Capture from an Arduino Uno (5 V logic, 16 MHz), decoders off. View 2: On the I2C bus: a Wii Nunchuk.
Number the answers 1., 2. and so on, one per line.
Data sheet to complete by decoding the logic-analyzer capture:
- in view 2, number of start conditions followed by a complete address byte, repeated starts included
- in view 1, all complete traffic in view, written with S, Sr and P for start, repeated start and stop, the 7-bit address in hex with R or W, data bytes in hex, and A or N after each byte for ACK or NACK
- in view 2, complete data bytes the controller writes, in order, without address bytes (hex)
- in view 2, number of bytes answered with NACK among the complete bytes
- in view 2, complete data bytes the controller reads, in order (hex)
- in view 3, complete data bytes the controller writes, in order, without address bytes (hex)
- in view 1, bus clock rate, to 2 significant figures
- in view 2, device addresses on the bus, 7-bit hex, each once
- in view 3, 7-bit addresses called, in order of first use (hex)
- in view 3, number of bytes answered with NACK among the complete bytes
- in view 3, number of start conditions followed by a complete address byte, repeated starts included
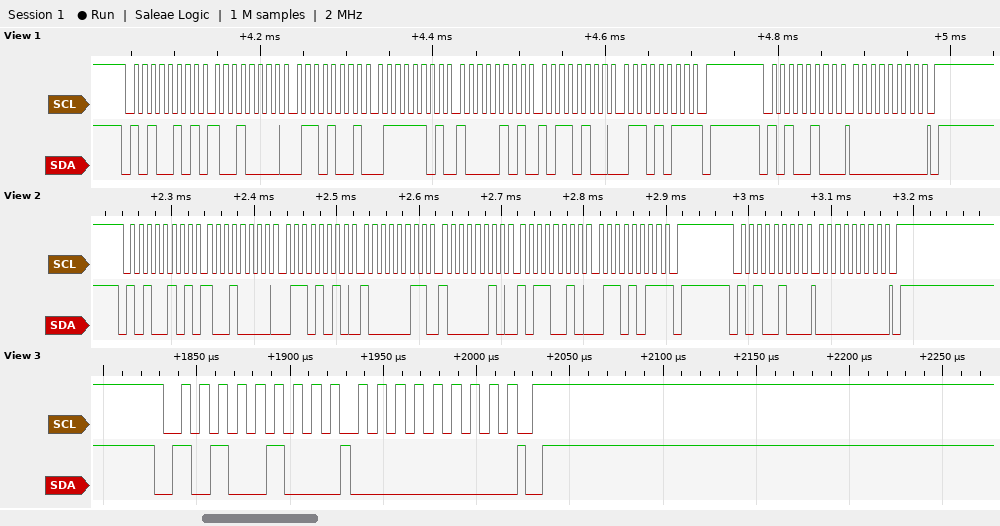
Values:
1. 2
2. S 52R A 90 A 69 A 7D A 85 A B4 A 6B N P S 52W A 00 A P
3. 00
4. 1
5. 90 6A 83 82 B2 6B
6. 00
7. 100 kHz
8. 0x52
9. 0x52
10. 0
11. 1
